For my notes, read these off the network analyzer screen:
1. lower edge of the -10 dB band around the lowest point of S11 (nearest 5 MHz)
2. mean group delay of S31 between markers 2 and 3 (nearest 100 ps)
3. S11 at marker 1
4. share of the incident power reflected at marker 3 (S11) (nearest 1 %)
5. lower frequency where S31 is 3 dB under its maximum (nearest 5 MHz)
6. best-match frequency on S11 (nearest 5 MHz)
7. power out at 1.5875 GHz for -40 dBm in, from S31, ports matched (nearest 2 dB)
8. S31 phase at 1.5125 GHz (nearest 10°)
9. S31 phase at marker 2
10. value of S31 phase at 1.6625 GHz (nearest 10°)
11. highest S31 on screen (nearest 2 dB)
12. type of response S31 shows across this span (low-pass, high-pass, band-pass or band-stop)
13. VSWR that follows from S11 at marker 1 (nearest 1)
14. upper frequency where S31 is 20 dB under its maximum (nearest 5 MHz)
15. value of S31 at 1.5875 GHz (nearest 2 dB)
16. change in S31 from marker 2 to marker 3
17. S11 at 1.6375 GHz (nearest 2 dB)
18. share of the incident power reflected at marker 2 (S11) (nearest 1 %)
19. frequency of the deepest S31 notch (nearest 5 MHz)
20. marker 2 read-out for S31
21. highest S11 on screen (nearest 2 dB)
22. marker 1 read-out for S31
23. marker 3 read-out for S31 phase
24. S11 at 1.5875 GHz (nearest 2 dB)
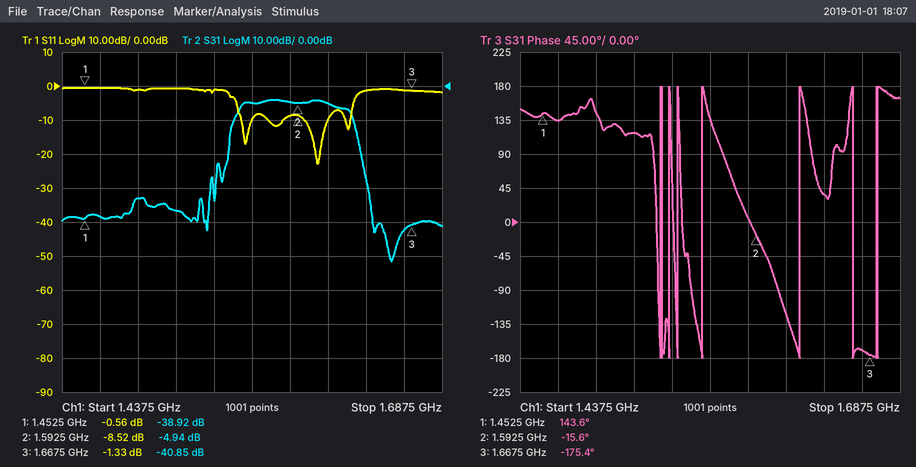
1.595 GHz
5.9 ns
-0.56 dB
74 %
1.555 GHz
1.605 GHz
-44 dBm
120°
-15.6°
-170°
-4 dB
band-pass
31
1.635 GHz
-4 dB
-35.91 dB
-2 dB
14 %
1.655 GHz
-4.94 dB
0 dB
-38.92 dB
-175.4°
-8 dB
